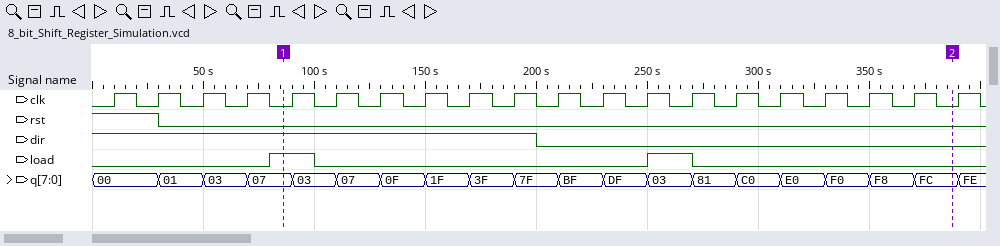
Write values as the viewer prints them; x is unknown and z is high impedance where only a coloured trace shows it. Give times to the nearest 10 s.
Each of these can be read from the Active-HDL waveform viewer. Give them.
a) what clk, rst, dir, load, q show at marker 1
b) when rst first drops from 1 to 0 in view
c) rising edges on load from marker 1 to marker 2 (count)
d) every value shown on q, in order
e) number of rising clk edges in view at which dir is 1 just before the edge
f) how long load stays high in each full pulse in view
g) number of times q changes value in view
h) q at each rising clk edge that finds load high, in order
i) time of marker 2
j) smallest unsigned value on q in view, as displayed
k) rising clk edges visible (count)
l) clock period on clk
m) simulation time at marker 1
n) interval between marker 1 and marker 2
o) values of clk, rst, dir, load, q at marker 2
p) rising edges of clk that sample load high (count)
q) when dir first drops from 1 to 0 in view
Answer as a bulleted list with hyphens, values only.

- clk=0, rst=0, dir=1, load=1, q=07
- 30 s
- 1
- 00, 01, 03, 07, 03, 07, 0F, 1F, 3F, 7F, BF, DF, 03, 81, C0, E0, F0, F8, FC, FE
- 10
- 20 s, 20 s
- 19
- 07, 03
- 390 s
- 00
- 20
- 20 s
- 90 s
- 300 s
- clk=0, rst=0, dir=0, load=0, q=FC
- 2
- 200 s
